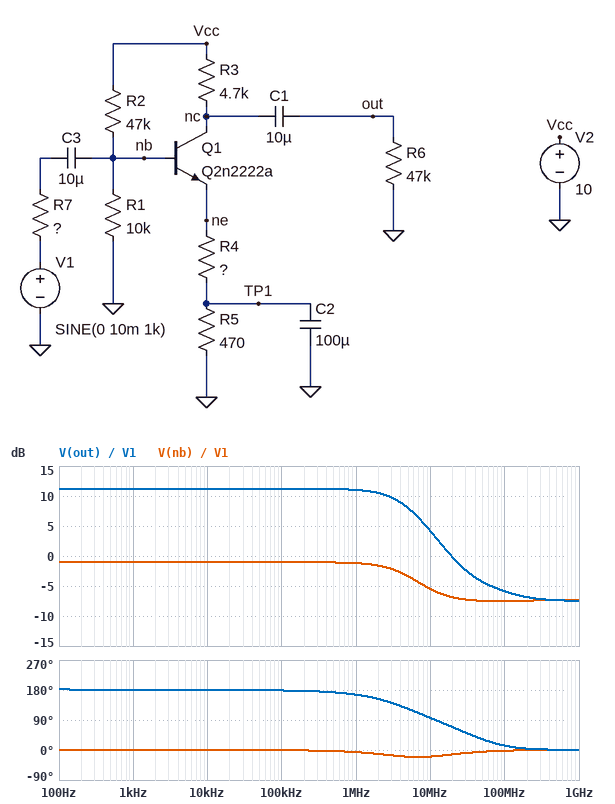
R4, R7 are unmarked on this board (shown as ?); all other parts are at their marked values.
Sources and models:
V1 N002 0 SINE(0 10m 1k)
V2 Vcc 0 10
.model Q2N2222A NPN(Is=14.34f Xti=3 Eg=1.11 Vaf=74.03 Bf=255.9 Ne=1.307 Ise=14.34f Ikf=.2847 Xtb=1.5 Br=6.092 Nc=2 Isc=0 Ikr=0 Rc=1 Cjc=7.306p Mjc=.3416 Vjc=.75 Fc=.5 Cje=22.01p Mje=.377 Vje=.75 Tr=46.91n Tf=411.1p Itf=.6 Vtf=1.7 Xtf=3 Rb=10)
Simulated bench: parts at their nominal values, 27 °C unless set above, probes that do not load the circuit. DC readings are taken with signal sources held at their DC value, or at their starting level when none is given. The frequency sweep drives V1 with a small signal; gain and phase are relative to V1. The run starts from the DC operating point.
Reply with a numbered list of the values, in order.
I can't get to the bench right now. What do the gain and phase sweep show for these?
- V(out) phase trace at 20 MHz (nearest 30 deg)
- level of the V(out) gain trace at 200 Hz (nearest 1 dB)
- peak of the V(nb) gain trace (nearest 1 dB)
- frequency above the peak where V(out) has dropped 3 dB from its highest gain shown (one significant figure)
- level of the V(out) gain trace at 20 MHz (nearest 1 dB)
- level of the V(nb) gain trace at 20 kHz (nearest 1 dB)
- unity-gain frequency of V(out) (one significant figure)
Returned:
1. 60 deg
2. 11 dB
3. -1 dB
4. 5 MHz
5. 0 dB
6. -1 dB
7. 20 MHz
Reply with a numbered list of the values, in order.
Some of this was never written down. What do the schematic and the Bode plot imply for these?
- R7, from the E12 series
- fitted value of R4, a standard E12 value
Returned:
1. 1 kΩ
2. 1 kΩ
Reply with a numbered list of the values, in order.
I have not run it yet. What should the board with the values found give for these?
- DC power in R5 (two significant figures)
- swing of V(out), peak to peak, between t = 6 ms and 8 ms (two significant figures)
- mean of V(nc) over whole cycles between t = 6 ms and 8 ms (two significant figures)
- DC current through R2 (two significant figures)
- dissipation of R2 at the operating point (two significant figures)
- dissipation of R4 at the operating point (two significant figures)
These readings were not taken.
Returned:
1. 250 µW
2. 73 mV
3. 6.6 V
4. 180 µA
5. 1.5 mW
6. 540 µW
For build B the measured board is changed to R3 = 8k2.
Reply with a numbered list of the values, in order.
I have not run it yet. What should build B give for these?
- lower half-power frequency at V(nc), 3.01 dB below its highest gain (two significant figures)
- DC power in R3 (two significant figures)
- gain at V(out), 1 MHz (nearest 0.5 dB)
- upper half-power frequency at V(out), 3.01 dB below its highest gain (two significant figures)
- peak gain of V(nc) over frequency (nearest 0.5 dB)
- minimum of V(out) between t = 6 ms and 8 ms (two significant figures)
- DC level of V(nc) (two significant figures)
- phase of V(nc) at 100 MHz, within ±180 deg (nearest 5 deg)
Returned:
1. 3.4 Hz
2. 4.3 mW
3. 15.0 dB
4. 2.5 MHz
5. 15.5 dB
6. -59 mV
7. 4.0 V
8. 10 deg
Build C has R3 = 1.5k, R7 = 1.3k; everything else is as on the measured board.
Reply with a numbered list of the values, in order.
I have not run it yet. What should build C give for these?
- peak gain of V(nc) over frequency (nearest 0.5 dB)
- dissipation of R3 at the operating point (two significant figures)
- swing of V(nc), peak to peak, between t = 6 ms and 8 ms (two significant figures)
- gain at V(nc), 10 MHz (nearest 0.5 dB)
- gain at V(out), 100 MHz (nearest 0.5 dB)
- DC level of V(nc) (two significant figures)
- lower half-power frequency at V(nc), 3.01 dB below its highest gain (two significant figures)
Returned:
1. 1.5 dB
2. 800 µW
3. 24 mV
4. -1.0 dB
5. -9.0 dB
6. 8.9 V
7. 3.3 Hz
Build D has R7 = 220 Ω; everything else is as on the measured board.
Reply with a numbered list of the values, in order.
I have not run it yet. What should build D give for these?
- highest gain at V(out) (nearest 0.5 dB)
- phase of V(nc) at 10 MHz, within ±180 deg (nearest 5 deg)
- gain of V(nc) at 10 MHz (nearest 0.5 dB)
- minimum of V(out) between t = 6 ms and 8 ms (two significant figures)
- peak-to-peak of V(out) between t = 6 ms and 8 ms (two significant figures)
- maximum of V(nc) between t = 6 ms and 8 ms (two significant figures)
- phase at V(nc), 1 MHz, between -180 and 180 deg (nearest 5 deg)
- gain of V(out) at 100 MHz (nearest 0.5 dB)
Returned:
1. 12.0 dB
2. 110 deg
3. 8.0 dB
4. -40 mV
5. 80 mV
6. 6.6 V
7. 170 deg
8. -0.5 dB
